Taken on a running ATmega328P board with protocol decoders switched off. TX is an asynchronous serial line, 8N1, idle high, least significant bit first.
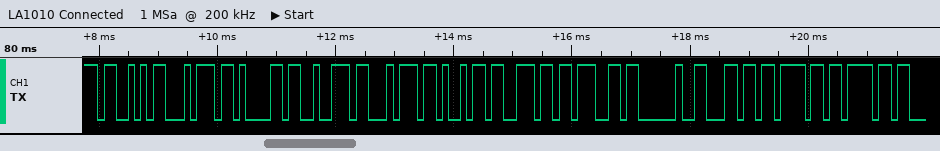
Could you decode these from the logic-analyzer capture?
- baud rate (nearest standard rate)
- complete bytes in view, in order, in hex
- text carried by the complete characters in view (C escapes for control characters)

9600 baud
53 74 61 72 74 69 6E 67 20 6C 6F 6F
"Starting loo"
